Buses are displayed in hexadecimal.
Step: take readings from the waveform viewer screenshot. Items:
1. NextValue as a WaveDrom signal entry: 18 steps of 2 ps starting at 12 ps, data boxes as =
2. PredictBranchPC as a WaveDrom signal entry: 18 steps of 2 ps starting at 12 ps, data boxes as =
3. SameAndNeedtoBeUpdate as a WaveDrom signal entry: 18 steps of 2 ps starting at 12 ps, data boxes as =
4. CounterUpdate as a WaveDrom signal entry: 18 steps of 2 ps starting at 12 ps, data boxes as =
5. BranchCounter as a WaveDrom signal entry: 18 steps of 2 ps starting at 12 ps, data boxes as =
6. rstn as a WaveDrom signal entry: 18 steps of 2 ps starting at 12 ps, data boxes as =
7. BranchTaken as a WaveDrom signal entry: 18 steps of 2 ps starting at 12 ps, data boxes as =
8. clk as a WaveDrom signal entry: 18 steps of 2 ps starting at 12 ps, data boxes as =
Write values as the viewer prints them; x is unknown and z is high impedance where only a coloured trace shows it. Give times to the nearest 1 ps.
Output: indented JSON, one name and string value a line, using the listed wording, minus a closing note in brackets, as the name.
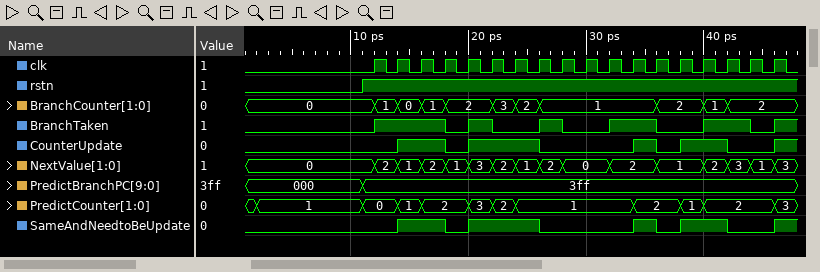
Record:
{
  "NextValue as a WaveDrom signal entry: 18 steps of 2 ps starting at 12 ps, data boxes as =": "{name: 'NextValue', wave: '=========.=.=.====', data: '2 1 2 1 3 2 1 2 0 2 1 2 3 1 3'}",
  "PredictBranchPC as a WaveDrom signal entry: 18 steps of 2 ps starting at 12 ps, data boxes as =": "{name: 'PredictBranchPC', wave: '=.................', data: '3ff'}",
  "SameAndNeedtoBeUpdate as a WaveDrom signal entry: 18 steps of 2 ps starting at 12 ps, data boxes as =": "{name: 'SameAndNeedtoBeUpdate', wave: '01.01..0...101.0.1'}",
  "CounterUpdate as a WaveDrom signal entry: 18 steps of 2 ps starting at 12 ps, data boxes as =": "{name: 'CounterUpdate', wave: '01.01..0...101.0.1'}",
  "BranchCounter as a WaveDrom signal entry: 18 steps of 2 ps starting at 12 ps, data boxes as =": "{name: 'BranchCounter', wave: '====.===....=.==..', data: '1 0 1 2 3 2 1 2 1 2'}",
  "rstn as a WaveDrom signal entry: 18 steps of 2 ps starting at 12 ps, data boxes as =": "{name: 'rstn', wave: '1.................'}",
  "BranchTaken as a WaveDrom signal entry: 18 steps of 2 ps starting at 12 ps, data boxes as =": "{name: 'BranchTaken', wave: '1..010.10.1.0.1.01'}",
  "clk as a WaveDrom signal entry: 18 steps of 2 ps starting at 12 ps, data boxes as =": "{name: 'clk', wave: 'p.................'}"
}
